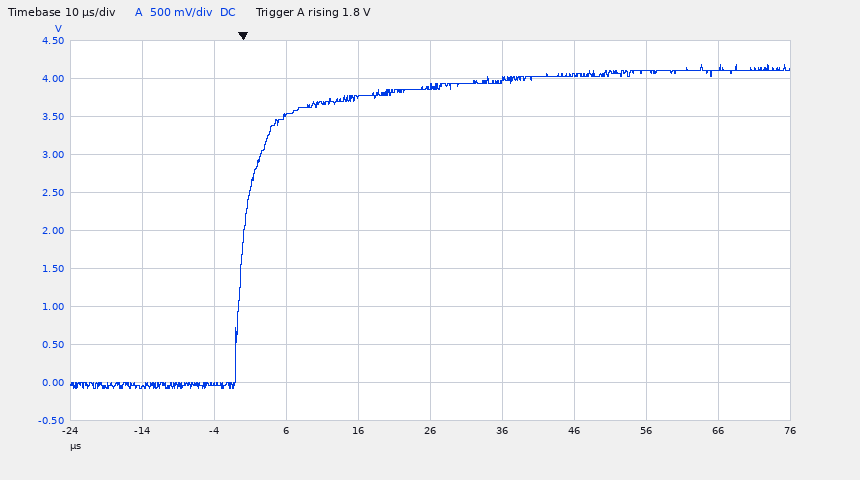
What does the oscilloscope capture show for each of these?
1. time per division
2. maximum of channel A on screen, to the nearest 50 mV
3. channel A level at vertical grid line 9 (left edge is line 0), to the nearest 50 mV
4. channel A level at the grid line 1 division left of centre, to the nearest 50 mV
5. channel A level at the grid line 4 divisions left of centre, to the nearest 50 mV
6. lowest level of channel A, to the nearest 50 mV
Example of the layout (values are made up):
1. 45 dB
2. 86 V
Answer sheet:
1. 10 µs
2. 4.20 V
3. 4.15 V
4. 3.75 V
5. -50 mV
6. -100 mV
